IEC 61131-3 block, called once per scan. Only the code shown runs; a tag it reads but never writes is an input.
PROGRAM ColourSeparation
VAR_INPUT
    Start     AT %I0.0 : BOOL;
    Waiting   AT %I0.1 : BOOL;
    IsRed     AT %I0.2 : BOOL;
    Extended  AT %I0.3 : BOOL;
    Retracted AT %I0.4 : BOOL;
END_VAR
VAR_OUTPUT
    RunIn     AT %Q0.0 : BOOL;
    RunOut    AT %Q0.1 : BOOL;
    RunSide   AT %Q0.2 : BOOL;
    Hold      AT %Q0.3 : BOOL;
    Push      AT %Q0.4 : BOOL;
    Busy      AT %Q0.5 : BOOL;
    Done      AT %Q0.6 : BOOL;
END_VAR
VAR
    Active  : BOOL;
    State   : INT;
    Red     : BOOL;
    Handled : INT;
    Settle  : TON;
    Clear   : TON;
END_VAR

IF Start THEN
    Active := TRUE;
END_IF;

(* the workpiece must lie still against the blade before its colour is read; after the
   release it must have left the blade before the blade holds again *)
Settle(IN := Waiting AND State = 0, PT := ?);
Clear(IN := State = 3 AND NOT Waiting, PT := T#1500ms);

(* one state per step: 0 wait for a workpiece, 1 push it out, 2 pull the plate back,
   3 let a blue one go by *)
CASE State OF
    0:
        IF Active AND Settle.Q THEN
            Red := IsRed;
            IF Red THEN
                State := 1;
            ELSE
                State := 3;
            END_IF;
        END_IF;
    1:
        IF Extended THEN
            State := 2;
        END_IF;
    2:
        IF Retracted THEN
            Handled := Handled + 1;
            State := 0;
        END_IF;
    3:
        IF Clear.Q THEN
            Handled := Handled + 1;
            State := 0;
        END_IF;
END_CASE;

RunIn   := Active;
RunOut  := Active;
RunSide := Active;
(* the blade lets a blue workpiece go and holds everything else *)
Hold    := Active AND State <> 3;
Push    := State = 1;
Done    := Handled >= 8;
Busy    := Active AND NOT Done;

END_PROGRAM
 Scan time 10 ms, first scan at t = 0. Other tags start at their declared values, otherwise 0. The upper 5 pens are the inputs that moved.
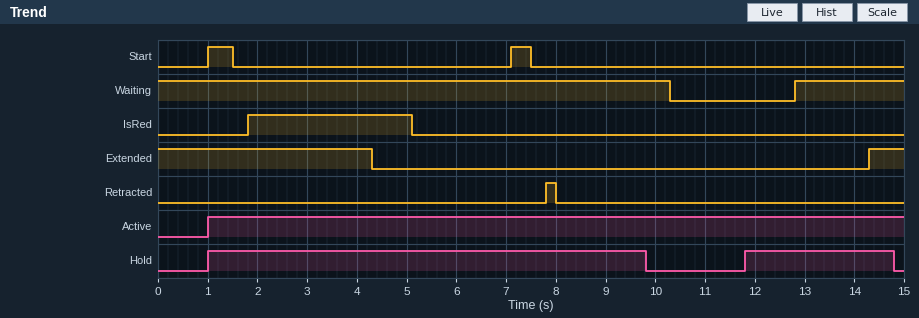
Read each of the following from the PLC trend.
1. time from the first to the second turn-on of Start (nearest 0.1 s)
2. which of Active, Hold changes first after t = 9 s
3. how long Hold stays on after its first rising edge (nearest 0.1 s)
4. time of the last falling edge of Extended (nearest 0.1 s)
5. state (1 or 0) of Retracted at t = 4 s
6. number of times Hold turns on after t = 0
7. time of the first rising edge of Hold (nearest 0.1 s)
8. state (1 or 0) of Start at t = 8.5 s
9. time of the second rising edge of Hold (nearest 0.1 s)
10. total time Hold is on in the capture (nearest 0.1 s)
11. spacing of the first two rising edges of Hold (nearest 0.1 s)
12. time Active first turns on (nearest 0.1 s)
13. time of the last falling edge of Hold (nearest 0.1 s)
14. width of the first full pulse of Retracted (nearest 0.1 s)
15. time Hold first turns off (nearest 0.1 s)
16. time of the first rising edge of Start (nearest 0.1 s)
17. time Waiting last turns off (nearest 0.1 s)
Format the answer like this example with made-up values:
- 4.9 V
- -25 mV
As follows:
- 6.1 s
- Hold
- 8.8 s
- 4.3 s
- 0
- 2
- 1.0 s
- 0
- 11.8 s
- 11.8 s
- 10.8 s
- 1.0 s
- 14.8 s
- 0.2 s
- 9.8 s
- 1.0 s
- 10.3 s
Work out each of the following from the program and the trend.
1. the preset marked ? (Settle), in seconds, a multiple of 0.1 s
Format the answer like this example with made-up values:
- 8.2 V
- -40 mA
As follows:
- 2.0 s
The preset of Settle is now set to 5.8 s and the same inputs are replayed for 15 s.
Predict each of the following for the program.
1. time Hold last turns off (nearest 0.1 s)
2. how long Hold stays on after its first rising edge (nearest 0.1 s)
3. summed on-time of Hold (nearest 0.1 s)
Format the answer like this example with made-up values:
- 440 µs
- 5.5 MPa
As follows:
- 5.8 s
- 4.8 s
- 8.0 s
